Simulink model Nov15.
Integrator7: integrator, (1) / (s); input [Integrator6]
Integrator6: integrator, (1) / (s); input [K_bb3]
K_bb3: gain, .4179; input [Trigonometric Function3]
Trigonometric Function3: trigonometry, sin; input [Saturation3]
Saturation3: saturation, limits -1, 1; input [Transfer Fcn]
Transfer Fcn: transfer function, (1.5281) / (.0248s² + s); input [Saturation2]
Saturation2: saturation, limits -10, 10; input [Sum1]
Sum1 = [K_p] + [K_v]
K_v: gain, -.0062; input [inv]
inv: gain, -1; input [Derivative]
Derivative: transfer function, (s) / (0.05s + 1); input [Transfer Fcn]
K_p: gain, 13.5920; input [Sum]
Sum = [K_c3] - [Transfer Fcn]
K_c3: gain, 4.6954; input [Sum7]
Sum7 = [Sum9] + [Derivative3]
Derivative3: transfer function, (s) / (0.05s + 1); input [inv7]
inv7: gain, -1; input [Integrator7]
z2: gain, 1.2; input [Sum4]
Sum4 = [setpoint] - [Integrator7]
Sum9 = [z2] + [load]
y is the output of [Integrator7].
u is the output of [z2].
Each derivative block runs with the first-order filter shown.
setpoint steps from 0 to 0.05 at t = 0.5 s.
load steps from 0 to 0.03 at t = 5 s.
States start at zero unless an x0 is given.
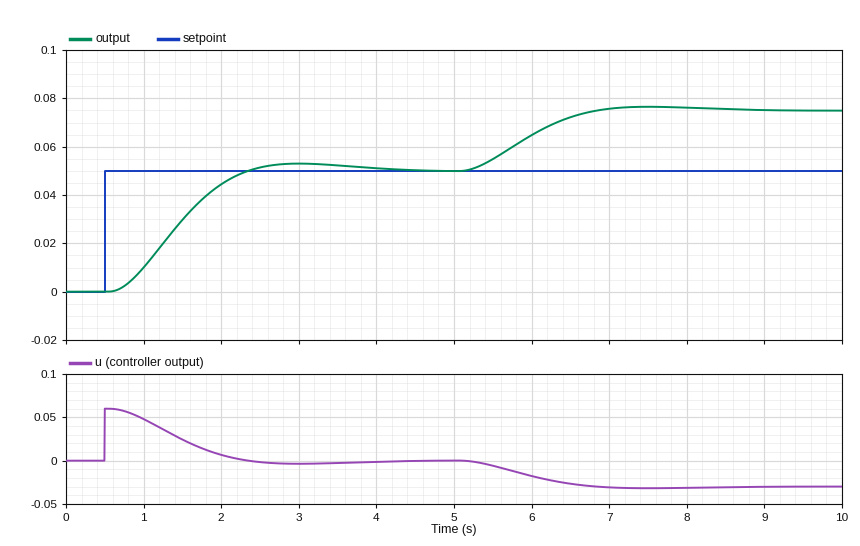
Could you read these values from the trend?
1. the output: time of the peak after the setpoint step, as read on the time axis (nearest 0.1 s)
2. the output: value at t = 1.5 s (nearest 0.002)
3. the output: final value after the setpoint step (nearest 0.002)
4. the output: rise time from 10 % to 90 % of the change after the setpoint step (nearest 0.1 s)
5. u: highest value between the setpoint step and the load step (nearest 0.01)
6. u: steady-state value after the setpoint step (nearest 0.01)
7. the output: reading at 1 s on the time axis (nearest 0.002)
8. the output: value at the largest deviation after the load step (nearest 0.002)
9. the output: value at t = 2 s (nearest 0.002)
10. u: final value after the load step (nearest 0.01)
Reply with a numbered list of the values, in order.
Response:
1. 3.0 s
2. 0.030
3. 0.050
4. 1.2 s
5. 0.06
6. 0.00
7. 0.010
8. 0.076
9. 0.044
10. -0.03
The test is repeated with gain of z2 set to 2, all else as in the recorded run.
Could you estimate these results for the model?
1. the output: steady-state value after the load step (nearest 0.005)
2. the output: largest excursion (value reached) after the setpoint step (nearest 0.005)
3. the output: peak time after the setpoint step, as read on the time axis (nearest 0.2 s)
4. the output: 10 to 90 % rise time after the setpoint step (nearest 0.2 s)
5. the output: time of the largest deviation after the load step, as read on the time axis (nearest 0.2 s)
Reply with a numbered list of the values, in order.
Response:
1. 0.065
2. 0.060
3. 2.2 s
4. 0.8 s
5. 6.6 s
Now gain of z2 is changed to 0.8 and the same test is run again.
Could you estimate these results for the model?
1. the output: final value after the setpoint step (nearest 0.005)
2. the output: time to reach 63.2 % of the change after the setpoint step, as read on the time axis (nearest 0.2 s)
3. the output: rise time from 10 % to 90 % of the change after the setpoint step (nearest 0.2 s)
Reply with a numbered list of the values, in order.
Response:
1. 0.050
2. 2.0 s
3. 1.8 s
